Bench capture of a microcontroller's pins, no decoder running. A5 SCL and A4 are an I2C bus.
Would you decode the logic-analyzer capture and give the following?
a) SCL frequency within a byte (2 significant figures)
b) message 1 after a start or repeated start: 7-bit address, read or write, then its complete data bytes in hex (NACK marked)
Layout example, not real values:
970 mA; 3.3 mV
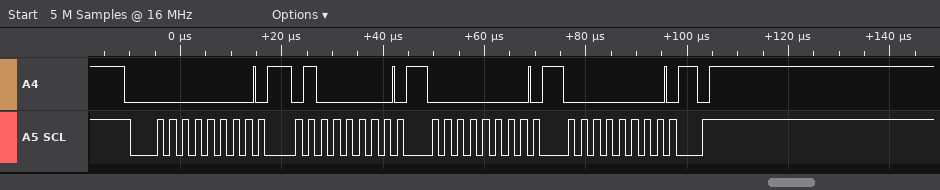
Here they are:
400 kHz; 0x00 write: 40 00 00
